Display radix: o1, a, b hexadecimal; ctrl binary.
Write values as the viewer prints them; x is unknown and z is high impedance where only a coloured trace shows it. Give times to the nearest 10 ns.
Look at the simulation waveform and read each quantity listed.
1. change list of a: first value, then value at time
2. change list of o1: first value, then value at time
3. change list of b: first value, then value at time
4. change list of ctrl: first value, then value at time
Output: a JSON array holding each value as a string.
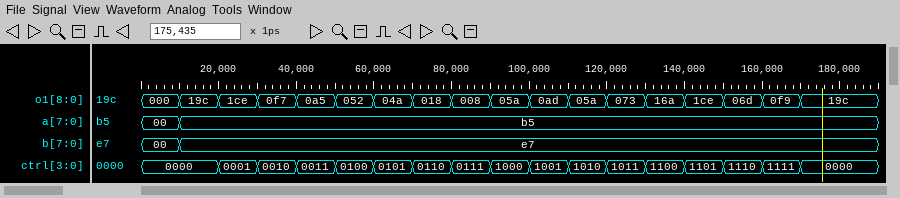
["00, b5 at 10 ns", "000, 19c at 10 ns, 1ce at 20 ns, 0f7 at 30 ns, 0a5 at 40 ns, 052 at 50 ns, 04a at 60 ns, 018 at 70 ns, 008 at 80 ns, 05a at 90 ns, 0ad at 100 ns, 05a at 110 ns, 073 at 120 ns, 16a at 130 ns, 1ce at 140 ns, 06d at 150 ns, 0f9 at 160 ns, 19c at 170 ns", "00, e7 at 10 ns", "0000, 0001 at 20 ns, 0010 at 30 ns, 0011 at 40 ns, 0100 at 50 ns, 0101 at 60 ns, 0110 at 70 ns, 0111 at 80 ns, 1000 at 90 ns, 1001 at 100 ns, 1010 at 110 ns, 1011 at 120 ns, 1100 at 130 ns, 1101 at 140 ns, 1110 at 150 ns, 1111 at 160 ns, 0000 at 170 ns"]
